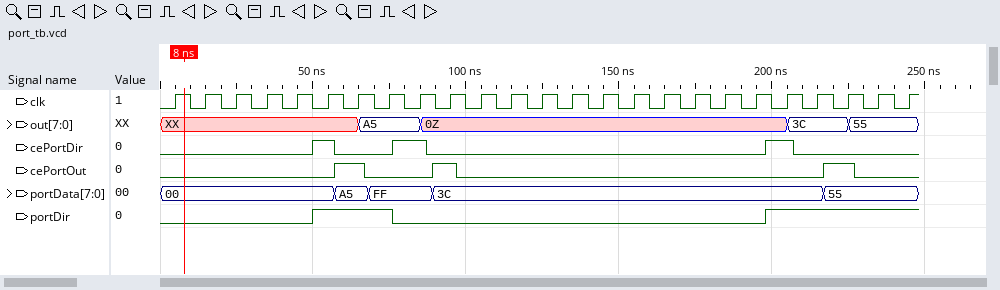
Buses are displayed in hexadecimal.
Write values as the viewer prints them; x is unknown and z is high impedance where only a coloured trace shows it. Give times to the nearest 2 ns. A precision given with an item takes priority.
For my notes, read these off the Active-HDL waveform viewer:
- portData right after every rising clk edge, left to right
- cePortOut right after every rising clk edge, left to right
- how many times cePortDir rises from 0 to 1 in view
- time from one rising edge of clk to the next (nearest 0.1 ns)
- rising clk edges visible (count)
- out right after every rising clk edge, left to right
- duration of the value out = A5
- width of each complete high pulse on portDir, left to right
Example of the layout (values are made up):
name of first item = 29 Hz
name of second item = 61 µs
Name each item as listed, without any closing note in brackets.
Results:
portData right after every rising clk edge, left to right = 00, 00, 00, 00, 00, 00, A5, FF, FF, 3C, 3C, 3C, 3C, 3C, 3C, 3C, 3C, 3C, 3C, 3C, 3C, 3C, 55, 55, 55
cePortOut right after every rising clk edge, left to right = 0 0 0 0 0 0 1 0 0 1 0 0 0 0 0 0 0 0 0 0 0 0 1 0 0
how many times cePortDir rises from 0 to 1 in view = 3
time from one rising edge of clk to the next = 10 ns
rising clk edges visible = 25
out right after every rising clk edge, left to right = XX, XX, XX, XX, XX, XX, A5, A5, 0Z, 0Z, 0Z, 0Z, 0Z, 0Z, 0Z, 0Z, 0Z, 0Z, 0Z, 0Z, 3C, 3C, 55, 55, 55
duration of the value out = A5 = 20 ns
width of each complete high pulse on portDir, left to right = 26 ns
